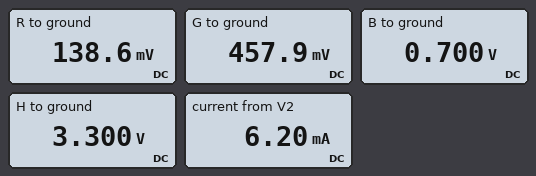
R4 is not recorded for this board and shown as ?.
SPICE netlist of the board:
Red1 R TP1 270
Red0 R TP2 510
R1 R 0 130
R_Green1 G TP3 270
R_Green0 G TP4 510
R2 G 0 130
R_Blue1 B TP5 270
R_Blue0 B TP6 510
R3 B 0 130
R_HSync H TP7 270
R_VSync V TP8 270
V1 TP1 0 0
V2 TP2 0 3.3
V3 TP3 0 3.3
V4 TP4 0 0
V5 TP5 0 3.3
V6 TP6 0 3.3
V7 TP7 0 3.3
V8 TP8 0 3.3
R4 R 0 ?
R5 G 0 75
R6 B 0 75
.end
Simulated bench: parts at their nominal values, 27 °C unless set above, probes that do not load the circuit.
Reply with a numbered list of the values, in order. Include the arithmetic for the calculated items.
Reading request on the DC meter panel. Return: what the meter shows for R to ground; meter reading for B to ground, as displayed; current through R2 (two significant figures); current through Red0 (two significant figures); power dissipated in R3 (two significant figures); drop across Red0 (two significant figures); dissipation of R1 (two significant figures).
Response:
1. 138.6 mV
2. 0.700 V
3. (457.9 mV) / 130 Ω = 3.5 mA
4. (3.3 V - 138.6 mV) / 510 Ω = 6.2 mA
5. (700 mV)^2 / 130 Ω = 3.8 mW
6. 3.3 V - 138.6 mV = 3.2 V
7. (138.6 mV)^2 / 130 Ω = 150 µW
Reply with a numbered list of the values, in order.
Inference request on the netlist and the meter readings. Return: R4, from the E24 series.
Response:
1. 30 Ω
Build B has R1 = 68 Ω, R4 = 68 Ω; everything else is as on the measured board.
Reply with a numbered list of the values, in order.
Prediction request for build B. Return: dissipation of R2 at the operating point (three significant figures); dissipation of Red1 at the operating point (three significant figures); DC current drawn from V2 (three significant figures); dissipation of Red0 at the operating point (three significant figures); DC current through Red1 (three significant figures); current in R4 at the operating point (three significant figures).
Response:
1. 1.61 mW
2. 126 µW
3. 6.11 mA
4. 19.0 mW
5. 683 µA
6. 2.71 mA
